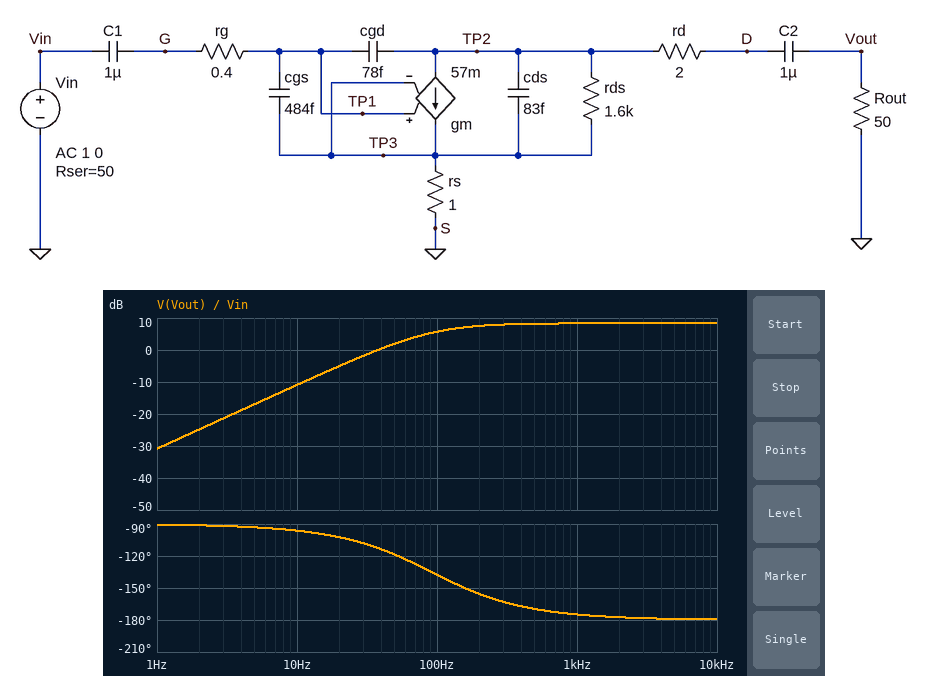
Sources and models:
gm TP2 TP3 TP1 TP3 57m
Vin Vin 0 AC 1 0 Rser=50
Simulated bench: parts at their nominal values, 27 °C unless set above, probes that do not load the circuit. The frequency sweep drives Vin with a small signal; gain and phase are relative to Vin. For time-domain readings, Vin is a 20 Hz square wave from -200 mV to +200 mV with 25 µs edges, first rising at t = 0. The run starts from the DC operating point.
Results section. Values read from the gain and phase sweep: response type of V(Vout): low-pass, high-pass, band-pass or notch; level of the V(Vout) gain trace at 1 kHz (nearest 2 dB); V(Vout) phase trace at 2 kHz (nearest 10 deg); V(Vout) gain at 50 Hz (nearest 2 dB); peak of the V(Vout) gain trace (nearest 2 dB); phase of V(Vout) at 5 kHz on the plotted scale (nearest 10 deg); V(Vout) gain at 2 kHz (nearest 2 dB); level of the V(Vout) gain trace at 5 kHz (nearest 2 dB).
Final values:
high-pass
8 dB
-180 deg
2 dB
8 dB
-180 deg
8 dB
8 dB
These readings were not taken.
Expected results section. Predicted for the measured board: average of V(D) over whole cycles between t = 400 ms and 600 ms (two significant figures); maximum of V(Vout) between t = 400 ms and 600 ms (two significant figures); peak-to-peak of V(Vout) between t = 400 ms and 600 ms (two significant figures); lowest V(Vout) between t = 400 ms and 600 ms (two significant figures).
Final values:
-18 V
1.0 V
2.1 V
-1.0 V
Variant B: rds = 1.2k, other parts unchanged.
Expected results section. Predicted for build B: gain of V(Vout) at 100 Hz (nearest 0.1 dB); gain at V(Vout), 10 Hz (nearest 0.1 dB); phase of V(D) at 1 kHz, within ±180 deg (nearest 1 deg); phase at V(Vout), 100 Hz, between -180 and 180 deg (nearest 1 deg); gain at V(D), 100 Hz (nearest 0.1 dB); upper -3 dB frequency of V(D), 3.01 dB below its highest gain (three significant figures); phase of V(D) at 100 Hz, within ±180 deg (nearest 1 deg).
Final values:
4.4 dB
-13.4 dB
114 deg
-130 deg
34.4 dB
121 Hz
142 deg
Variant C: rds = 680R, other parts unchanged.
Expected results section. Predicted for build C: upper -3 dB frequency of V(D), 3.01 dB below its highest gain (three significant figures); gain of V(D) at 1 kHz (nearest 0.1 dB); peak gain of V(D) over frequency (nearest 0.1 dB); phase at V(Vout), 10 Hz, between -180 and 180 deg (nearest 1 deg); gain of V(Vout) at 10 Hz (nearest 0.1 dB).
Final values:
207 Hz
18.3 dB
31.8 dB
-93 deg
-18.3 dB
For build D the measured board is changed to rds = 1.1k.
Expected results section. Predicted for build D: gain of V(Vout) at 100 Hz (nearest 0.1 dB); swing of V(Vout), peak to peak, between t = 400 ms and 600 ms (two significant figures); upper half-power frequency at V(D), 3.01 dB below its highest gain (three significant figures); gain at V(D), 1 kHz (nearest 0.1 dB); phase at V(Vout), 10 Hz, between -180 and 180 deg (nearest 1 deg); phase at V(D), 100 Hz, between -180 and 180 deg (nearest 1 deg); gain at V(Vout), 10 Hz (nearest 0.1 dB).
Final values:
3.9 dB
2.0 V
131 Hz
18.6 dB
-94 deg
144 deg
-14.1 dB
